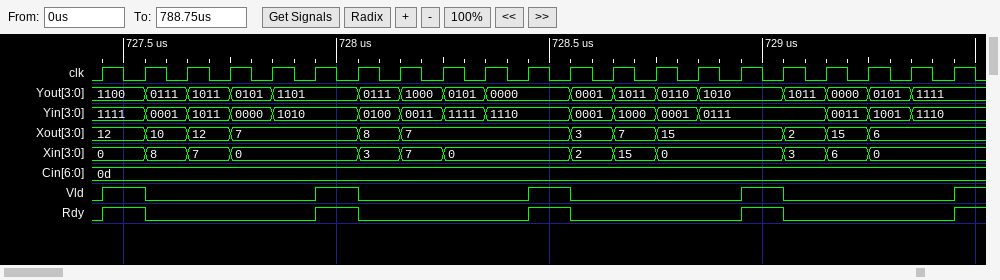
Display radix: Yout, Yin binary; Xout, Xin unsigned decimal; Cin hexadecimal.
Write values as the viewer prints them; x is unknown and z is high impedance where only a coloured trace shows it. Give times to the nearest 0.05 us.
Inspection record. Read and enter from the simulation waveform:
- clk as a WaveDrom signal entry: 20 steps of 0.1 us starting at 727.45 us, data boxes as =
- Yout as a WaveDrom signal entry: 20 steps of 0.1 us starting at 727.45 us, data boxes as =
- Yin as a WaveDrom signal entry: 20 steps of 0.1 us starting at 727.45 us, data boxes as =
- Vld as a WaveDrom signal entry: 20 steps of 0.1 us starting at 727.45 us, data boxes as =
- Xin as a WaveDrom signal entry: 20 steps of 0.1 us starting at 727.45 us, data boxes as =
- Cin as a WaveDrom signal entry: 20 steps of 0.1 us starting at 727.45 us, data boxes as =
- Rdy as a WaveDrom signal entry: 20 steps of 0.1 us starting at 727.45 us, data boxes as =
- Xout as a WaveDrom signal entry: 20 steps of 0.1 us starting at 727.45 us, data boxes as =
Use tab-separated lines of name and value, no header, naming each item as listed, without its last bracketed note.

clk as a WaveDrom signal entry: 20 steps of 0.1 us starting at 727.45 us, data boxes as =	{name: 'clk', wave: 'p...................'}
Yout as a WaveDrom signal entry: 20 steps of 0.1 us starting at 727.45 us, data boxes as =	{name: 'Yout', wave: '=====.====.====.====', data: '1100 0111 1011 0101 1101 0111 1000 0101 0000 0001 1011 0110 1010 1011 0000 0101 1111'}
Yin as a WaveDrom signal entry: 20 steps of 0.1 us starting at 727.45 us, data boxes as =	{name: 'Yin', wave: '=====.====.====..===', data: '1111 0001 1011 0000 1010 0100 0011 1111 1110 0001 1000 0001 0111 0011 1001 1110'}
Vld as a WaveDrom signal entry: 20 steps of 0.1 us starting at 727.45 us, data boxes as =	{name: 'Vld', wave: '10...10...10...10...'}
Xin as a WaveDrom signal entry: 20 steps of 0.1 us starting at 727.45 us, data boxes as =	{name: 'Xin', wave: '====..===..===..===.', data: '0 8 7 0 3 7 0 2 15 0 3 6 0'}
Cin as a WaveDrom signal entry: 20 steps of 0.1 us starting at 727.45 us, data boxes as =	{name: 'Cin', wave: '=...................', data: '0d'}
Rdy as a WaveDrom signal entry: 20 steps of 0.1 us starting at 727.45 us, data boxes as =	{name: 'Rdy', wave: '10...10...10...10...'}
Xout as a WaveDrom signal entry: 20 steps of 0.1 us starting at 727.45 us, data boxes as =	{name: 'Xout', wave: '====..==...===..===.', data: '12 10 12 7 8 7 3 7 15 2 15 6'}
